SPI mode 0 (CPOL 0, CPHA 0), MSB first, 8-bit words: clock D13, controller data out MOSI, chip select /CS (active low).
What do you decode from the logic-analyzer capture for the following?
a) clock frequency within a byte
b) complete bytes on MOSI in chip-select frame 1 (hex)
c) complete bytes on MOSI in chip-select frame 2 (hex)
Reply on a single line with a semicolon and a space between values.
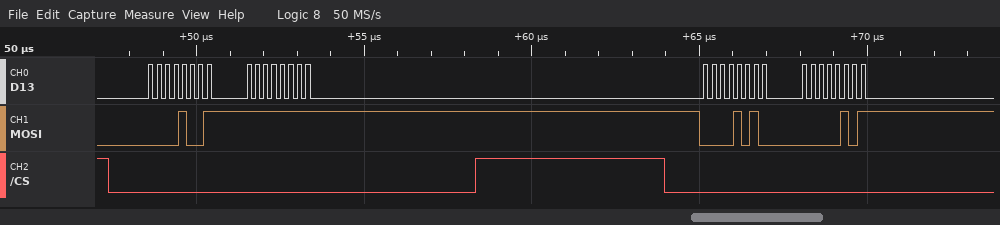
4 MHz; 09 FF; 0A 05
